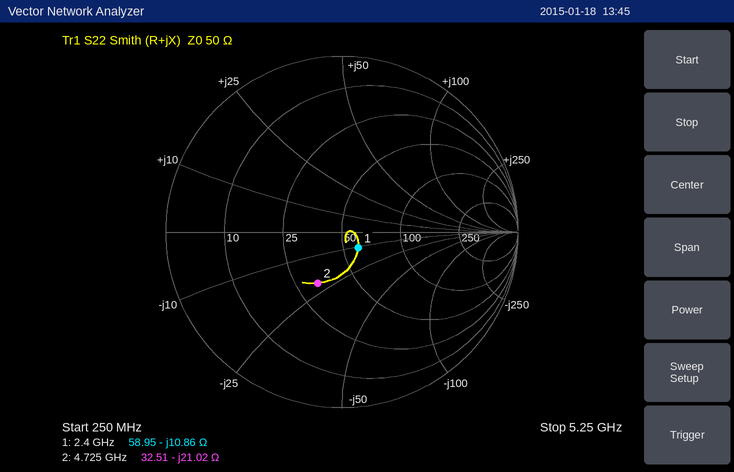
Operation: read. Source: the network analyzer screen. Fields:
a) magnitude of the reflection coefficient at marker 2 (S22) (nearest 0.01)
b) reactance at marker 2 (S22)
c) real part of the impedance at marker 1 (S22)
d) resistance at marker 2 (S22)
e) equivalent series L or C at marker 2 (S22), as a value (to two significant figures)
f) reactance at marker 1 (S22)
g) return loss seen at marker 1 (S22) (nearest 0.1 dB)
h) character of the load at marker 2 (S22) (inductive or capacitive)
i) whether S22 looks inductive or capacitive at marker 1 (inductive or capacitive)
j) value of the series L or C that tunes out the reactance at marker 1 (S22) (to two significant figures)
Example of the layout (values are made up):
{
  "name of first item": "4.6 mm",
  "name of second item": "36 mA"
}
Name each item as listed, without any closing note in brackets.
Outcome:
{
  "magnitude of the reflection coefficient at marker 2 (S22)": "0.32",
  "reactance at marker 2": "-21.02 Ω",
  "real part of the impedance at marker 1": "58.95 Ω",
  "resistance at marker 2": "32.51 Ω",
  "equivalent series L or C at marker 2 (S22), as a value": "1.6 pF",
  "reactance at marker 1": "-10.86 Ω",
  "return loss seen at marker 1 (S22)": "17.8 dB",
  "character of the load at marker 2 (S22)": "capacitive",
  "whether S22 looks inductive or capacitive at marker 1": "capacitive",
  "value of the series L or C that tunes out the reactance at marker 1 (S22)": "720 pH"
}
